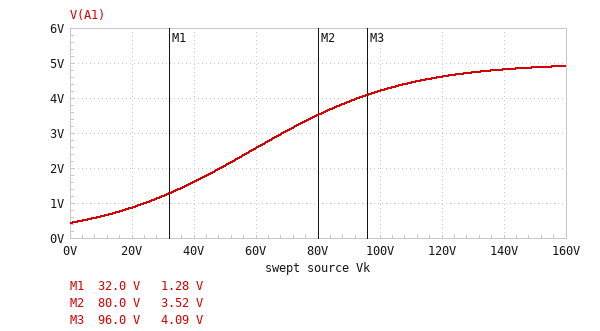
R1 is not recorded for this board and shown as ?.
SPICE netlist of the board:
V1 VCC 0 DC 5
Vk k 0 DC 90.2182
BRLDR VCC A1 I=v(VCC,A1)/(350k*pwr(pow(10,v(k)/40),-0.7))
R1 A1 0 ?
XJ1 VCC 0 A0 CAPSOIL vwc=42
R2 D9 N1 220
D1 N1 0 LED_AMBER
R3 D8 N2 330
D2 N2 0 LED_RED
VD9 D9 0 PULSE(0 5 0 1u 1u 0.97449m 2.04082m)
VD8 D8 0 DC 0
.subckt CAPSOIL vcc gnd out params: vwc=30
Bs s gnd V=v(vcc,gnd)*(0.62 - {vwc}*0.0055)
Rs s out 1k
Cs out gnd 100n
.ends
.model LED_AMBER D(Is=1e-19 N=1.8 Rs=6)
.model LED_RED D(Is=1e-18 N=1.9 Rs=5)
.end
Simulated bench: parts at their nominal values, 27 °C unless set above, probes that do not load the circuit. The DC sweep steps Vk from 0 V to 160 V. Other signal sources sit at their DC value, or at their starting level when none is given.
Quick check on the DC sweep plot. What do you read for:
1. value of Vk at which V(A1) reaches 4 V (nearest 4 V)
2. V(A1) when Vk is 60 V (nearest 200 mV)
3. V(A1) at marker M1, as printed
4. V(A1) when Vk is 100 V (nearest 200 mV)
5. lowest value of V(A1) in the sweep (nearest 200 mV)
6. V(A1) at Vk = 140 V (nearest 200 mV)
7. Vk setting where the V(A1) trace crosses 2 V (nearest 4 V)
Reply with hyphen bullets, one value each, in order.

- 92 V
- 2.6 V
- 1.28 V
- 4.2 V
- 400 mV
- 4.8 V
- 48 V
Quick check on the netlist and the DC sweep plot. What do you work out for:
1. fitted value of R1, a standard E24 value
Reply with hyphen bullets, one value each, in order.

- 33 kΩ
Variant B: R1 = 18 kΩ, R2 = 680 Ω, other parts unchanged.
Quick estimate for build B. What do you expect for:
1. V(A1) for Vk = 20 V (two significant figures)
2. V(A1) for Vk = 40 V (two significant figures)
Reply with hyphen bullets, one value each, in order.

- 520 mV
- 1.0 V
